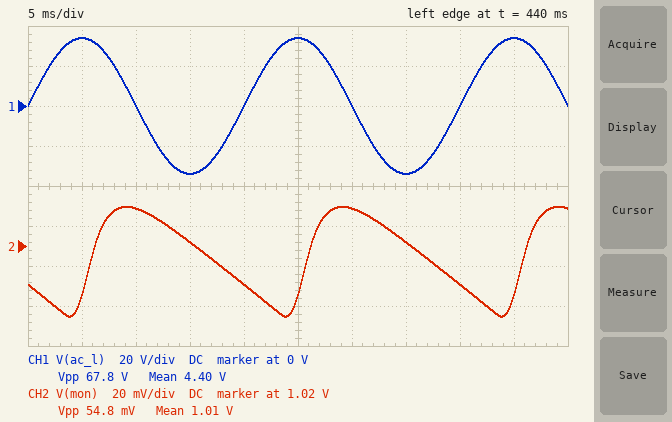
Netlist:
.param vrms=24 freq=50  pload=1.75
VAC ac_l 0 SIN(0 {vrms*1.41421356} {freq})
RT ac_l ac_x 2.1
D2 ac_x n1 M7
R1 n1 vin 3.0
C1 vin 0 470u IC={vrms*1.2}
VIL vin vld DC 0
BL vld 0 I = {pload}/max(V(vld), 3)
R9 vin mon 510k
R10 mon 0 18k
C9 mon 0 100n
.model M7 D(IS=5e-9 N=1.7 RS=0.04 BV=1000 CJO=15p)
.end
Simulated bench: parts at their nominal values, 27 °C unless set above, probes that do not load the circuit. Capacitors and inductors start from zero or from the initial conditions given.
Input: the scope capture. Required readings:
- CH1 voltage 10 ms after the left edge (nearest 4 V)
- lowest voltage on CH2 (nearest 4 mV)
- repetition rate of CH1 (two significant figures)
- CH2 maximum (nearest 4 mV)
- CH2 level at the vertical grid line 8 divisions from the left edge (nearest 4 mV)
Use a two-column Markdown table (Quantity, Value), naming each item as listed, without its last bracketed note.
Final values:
| Quantity | Value |
|---|---|
| CH1 voltage 10 ms after the left edge | 0 V |
| lowest voltage on CH2 | 984 mV |
| repetition rate of CH1 | 50 Hz |
| CH2 maximum | 1.040 V |
| CH2 level at the vertical grid line 8 divisions from the left edge | 1.000 V |
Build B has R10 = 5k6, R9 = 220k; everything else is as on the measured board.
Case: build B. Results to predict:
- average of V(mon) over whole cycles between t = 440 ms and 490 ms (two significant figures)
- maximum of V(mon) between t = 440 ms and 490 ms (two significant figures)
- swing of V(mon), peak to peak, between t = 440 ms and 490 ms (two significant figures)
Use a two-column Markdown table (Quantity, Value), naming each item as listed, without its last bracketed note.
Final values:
| Quantity | Value |
|---|---|
| average of V(mon) over whole cycles between t = 440 ms and 490 ms | 740 mV |
| maximum of V(mon) between t = 440 ms and 490 ms | 760 mV |
| swing of V(mon), peak to peak, between t = 440 ms and 490 ms | 50 mV |
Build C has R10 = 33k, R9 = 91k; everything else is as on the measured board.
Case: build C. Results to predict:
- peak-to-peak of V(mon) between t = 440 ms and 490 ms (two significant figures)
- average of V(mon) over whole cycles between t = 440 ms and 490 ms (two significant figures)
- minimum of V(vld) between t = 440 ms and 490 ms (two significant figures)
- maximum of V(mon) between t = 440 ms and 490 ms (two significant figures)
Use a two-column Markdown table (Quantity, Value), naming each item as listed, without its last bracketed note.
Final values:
| Quantity | Value |
|---|---|
| peak-to-peak of V(mon) between t = 440 ms and 490 ms | 380 mV |
| average of V(mon) over whole cycles between t = 440 ms and 490 ms | 7.9 V |
| minimum of V(vld) between t = 440 ms and 490 ms | 29 V |
| maximum of V(mon) between t = 440 ms and 490 ms | 8.1 V |
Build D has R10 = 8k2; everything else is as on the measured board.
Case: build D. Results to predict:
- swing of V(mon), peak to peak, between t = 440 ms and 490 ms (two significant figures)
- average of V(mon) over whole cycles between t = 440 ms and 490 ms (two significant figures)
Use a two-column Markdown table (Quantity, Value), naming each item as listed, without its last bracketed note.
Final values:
| Quantity | Value |
|---|---|
| swing of V(mon), peak to peak, between t = 440 ms and 490 ms | 30 mV |
| average of V(mon) over whole cycles between t = 440 ms and 490 ms | 470 mV |
